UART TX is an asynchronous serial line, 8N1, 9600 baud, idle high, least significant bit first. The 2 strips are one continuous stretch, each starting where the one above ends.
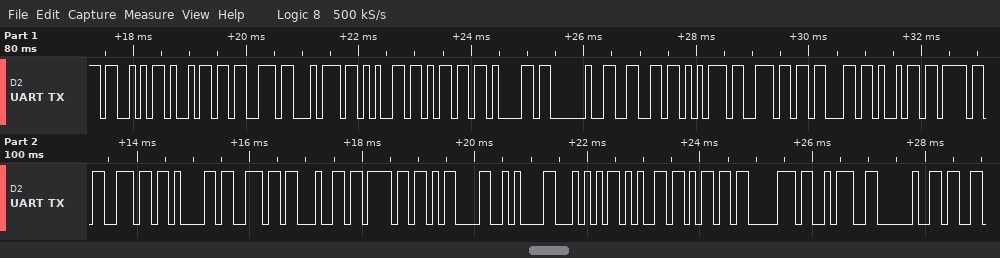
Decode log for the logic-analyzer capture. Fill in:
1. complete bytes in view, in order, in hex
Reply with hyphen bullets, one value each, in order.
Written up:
- 53 69 73 74 65 6D 61 20 66 75 6E 63 69 6F 6E 61 6E 64 6F 0D 0A 54 65 6D 70 3A 20
